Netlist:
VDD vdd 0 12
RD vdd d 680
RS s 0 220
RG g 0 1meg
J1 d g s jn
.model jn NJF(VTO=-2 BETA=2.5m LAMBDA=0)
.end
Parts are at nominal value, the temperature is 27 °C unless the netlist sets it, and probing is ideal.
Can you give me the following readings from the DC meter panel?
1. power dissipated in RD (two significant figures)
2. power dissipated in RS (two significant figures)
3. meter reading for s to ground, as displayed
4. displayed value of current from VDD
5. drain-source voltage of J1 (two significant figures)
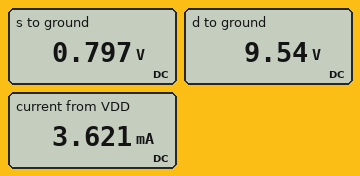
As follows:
8.9 mW
2.9 mW
0.797 V
3.621 mA
8.7 V
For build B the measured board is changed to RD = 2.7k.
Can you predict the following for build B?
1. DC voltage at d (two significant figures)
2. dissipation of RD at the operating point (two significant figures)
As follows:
2.2 V
35 mW
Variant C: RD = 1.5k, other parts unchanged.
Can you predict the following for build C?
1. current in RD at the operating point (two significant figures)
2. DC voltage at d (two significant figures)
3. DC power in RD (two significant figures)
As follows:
3.6 mA
6.6 V
20 mW
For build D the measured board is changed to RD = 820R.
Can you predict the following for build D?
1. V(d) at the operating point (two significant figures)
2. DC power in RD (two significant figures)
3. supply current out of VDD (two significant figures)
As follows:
9.0 V
11 mW
3.6 mA
